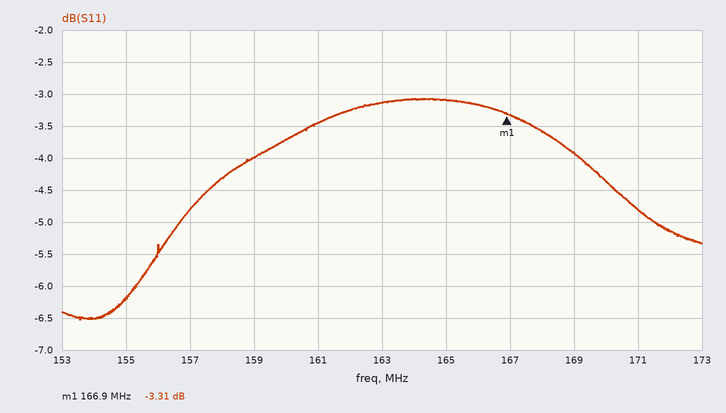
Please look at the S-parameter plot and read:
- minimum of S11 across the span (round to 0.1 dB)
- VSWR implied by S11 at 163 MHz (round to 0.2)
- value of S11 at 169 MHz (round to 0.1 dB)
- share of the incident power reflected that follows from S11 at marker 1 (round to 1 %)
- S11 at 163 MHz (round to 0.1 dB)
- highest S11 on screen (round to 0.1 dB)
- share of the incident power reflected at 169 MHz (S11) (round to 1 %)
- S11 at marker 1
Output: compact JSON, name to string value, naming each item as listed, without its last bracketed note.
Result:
{"minimum of S11 across the span": "-6.5 dB", "VSWR implied by S11 at 163 MHz": "5.6", "value of S11 at 169 MHz": "-3.9 dB", "share of the incident power reflected that follows from S11 at marker 1": "47 %", "S11 at 163 MHz": "-3.1 dB", "highest S11 on screen": "-3.1 dB", "share of the incident power reflected at 169 MHz (S11)": "41 %", "S11 at marker 1": "-3.31 dB"}
